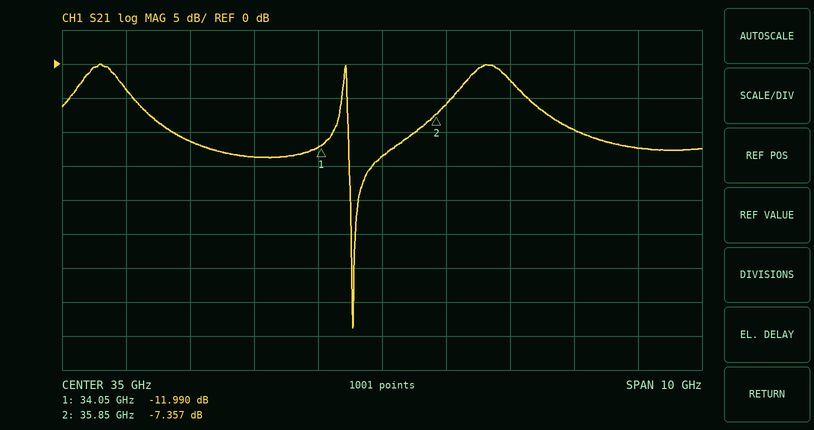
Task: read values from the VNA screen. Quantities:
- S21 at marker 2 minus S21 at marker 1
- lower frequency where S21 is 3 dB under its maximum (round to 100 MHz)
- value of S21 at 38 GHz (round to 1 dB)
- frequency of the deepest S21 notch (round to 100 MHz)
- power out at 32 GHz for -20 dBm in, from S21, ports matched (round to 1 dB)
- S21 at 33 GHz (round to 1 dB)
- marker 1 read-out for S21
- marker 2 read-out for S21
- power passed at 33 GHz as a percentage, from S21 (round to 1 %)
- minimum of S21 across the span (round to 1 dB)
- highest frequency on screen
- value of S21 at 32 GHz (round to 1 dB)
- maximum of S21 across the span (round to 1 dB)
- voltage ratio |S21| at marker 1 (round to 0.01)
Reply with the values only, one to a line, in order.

4.633 dB
30.3 GHz
-10 dB
34.5 GHz
-31 dBm
-14 dB
-11.990 dB
-7.357 dB
4 %
-39 dB
40 GHz
-11 dB
0 dB
0.25
